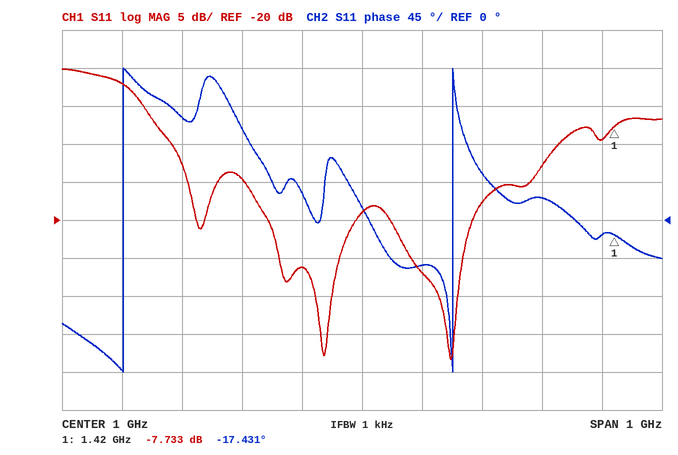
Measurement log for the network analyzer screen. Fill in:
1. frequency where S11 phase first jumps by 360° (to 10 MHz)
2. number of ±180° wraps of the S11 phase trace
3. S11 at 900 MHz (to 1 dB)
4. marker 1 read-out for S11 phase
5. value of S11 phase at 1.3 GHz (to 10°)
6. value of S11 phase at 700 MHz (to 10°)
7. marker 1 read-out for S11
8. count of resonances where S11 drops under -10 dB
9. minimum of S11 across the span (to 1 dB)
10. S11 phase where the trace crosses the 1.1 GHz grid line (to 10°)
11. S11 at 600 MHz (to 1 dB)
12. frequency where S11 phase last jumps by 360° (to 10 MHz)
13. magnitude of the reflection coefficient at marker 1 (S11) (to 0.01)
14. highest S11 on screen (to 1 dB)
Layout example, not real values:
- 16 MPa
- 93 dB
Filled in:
- 600 MHz
- 2
- -26 dB
- -17.431°
- 30°
- 120°
- -7.733 dB
- 3
- -38 dB
- -50°
- -2 dB
- 1.15 GHz
- 0.41
- 0 dB
